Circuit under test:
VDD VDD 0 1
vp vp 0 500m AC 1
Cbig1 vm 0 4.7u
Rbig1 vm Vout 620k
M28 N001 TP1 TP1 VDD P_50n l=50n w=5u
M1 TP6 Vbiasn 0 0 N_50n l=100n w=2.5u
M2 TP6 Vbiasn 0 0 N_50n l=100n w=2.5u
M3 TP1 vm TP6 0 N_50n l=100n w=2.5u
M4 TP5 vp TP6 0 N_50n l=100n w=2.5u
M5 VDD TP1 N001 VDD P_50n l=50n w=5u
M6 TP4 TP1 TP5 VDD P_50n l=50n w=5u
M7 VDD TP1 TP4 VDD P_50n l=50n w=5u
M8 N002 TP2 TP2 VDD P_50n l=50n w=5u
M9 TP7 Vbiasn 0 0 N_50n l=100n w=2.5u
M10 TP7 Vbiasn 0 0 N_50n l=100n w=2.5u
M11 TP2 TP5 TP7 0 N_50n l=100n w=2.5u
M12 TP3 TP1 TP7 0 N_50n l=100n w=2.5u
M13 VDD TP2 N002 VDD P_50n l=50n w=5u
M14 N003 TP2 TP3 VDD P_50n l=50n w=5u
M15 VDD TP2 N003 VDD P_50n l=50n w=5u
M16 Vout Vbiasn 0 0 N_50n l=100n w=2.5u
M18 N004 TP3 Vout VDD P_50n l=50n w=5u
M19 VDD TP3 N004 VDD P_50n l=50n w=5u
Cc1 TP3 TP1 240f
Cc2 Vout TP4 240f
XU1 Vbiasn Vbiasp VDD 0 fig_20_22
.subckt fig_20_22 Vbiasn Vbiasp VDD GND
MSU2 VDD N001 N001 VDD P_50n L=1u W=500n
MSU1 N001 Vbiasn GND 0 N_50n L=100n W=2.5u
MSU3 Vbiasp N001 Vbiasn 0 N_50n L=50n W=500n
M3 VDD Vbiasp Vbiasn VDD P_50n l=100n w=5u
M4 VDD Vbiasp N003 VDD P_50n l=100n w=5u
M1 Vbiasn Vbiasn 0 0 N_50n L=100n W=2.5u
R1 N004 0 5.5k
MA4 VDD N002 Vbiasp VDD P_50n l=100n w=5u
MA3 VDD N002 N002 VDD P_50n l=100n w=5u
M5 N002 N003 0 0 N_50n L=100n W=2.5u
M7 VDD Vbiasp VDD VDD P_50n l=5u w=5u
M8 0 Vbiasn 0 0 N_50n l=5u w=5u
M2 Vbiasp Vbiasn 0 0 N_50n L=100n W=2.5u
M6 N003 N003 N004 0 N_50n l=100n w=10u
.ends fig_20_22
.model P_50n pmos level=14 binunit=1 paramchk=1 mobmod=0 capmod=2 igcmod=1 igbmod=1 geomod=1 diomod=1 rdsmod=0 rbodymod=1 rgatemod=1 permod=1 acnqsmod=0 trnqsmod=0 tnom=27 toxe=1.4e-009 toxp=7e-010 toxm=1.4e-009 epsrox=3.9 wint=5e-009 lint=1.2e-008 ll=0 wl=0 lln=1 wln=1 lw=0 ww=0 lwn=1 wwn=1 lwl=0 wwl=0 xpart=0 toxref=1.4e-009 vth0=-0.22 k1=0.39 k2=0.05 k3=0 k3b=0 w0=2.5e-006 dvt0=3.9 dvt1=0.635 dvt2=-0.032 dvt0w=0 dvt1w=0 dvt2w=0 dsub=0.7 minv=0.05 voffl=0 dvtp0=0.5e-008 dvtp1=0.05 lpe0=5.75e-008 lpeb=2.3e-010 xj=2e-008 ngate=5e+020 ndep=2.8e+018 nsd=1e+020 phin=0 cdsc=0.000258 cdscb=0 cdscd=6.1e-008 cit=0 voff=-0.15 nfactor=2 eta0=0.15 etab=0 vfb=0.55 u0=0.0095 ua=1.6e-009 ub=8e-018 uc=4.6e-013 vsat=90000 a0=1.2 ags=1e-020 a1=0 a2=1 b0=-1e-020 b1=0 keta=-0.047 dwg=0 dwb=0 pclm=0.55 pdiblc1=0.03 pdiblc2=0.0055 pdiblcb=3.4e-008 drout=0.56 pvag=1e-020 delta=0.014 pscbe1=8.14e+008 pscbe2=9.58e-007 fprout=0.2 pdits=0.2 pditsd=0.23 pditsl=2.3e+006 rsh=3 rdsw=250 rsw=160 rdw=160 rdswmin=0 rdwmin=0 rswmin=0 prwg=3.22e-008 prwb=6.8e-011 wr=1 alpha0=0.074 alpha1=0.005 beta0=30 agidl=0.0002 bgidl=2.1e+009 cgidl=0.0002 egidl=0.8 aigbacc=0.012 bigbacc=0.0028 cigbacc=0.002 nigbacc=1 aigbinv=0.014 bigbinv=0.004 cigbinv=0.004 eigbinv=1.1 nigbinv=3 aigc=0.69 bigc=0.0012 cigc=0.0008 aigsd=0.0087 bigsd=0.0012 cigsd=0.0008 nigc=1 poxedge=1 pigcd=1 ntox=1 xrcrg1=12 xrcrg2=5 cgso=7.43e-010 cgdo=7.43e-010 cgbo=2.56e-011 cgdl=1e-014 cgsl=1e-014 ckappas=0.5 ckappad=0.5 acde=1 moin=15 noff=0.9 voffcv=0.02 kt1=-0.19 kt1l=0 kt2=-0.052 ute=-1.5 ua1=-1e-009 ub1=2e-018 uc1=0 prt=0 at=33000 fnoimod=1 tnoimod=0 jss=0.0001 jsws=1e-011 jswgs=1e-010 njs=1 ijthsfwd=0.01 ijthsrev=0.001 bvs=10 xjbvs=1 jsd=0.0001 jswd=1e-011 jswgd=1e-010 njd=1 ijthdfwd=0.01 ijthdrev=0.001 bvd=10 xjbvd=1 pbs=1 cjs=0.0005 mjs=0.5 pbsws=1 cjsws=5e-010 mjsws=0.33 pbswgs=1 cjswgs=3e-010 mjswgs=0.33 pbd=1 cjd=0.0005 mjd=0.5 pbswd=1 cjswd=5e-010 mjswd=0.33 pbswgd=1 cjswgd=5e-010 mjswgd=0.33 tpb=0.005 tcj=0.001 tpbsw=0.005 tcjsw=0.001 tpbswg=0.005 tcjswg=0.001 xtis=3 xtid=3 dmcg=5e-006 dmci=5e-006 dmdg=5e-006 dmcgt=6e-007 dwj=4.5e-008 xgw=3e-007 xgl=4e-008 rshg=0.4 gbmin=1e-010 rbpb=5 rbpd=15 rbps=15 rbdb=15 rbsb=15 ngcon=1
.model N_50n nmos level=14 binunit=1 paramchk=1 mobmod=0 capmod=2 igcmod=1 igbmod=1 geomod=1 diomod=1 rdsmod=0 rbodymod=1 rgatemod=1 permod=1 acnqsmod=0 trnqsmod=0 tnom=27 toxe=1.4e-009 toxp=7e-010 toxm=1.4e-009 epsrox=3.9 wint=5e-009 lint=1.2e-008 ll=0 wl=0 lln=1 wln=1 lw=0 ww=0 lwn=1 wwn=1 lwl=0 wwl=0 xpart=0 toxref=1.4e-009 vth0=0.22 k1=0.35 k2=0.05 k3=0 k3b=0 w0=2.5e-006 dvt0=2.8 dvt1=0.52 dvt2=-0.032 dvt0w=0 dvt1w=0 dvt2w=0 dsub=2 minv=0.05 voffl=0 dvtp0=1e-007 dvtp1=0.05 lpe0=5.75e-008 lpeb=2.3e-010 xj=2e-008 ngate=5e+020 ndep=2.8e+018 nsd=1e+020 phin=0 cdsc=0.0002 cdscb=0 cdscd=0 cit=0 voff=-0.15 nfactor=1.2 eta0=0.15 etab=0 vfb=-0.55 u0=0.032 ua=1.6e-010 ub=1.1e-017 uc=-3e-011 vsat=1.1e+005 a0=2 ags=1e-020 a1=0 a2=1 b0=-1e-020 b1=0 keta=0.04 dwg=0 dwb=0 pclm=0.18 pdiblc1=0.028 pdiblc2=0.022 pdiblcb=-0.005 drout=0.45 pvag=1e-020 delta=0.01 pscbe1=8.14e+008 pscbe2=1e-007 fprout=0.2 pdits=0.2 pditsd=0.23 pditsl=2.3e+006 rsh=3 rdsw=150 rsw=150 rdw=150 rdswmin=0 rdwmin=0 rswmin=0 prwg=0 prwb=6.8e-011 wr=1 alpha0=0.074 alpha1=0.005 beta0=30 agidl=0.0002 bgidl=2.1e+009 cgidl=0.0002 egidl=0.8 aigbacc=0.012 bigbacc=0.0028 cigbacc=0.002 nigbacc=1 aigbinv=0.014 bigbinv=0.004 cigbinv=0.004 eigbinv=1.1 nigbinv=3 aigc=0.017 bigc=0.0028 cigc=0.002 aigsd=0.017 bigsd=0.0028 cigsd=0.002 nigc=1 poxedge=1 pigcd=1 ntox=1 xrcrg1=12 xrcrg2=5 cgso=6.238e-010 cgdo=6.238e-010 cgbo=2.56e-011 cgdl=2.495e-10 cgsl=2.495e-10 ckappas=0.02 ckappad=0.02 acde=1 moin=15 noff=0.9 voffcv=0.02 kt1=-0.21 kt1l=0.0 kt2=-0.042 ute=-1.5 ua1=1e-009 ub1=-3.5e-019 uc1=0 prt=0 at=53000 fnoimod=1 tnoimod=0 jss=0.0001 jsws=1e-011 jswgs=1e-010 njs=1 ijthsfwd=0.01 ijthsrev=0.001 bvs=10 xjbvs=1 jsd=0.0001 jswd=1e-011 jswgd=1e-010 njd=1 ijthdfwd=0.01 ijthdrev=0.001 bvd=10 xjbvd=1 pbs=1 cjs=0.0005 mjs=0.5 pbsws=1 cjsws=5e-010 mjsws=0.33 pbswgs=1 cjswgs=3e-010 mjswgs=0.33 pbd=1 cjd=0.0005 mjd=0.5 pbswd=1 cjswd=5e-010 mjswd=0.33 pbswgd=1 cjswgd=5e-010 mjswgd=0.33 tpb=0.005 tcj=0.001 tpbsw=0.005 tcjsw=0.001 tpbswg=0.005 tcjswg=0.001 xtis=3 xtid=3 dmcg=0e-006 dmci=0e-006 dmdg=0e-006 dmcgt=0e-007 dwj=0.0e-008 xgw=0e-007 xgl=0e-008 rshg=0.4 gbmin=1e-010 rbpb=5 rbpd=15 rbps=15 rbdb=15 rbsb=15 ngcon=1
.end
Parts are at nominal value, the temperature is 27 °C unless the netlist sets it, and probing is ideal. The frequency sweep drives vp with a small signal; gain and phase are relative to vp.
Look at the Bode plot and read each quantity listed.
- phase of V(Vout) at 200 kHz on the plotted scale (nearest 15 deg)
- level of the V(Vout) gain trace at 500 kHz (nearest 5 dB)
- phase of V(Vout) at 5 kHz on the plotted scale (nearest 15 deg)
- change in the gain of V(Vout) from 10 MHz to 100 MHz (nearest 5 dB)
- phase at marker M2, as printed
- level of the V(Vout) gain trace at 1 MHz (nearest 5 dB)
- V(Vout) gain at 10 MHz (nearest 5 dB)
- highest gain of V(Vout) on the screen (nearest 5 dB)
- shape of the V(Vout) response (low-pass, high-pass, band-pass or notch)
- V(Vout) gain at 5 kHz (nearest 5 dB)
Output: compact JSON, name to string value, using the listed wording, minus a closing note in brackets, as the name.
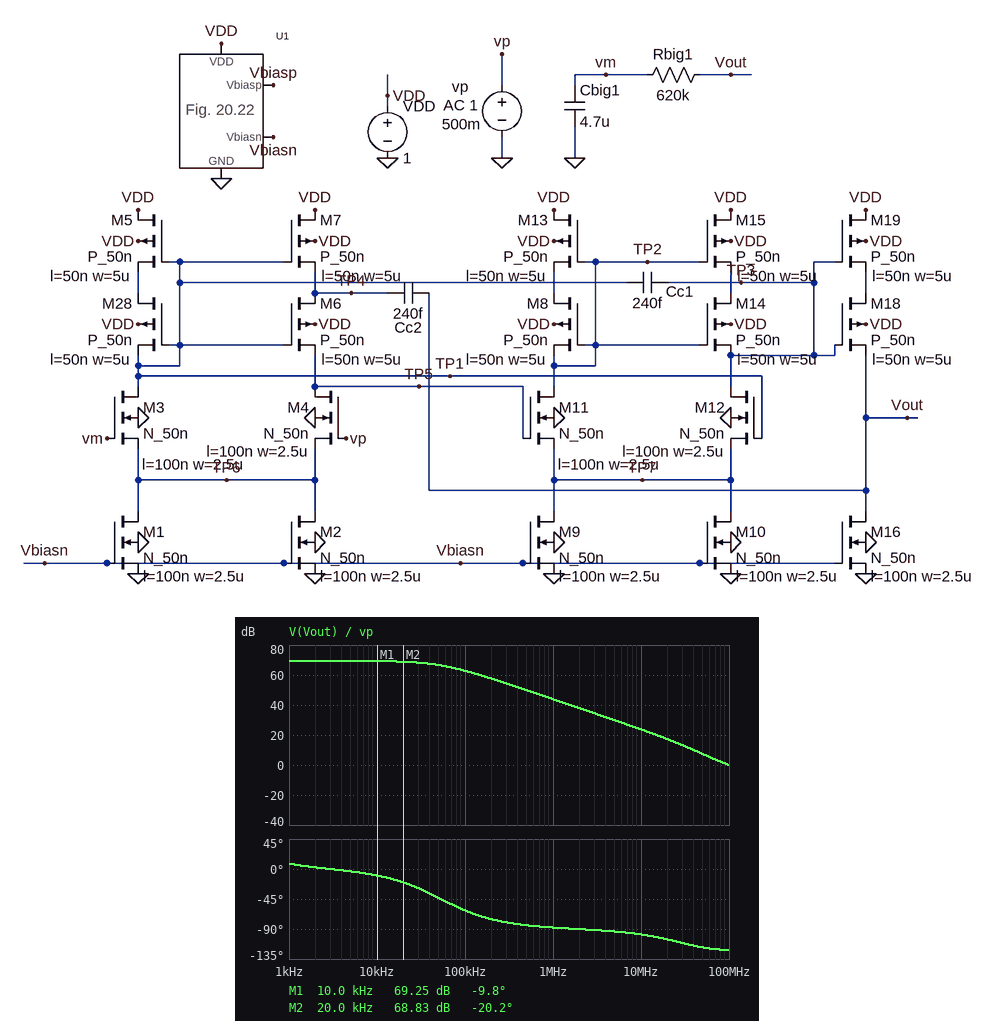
{"phase of V(Vout) at 200 kHz on the plotted scale": "-75 deg", "level of the V(Vout) gain trace at 500 kHz": "50 dB", "phase of V(Vout) at 5 kHz on the plotted scale": "0 deg", "change in the gain of V(Vout) from 10 MHz to 100 MHz": "-25 dB", "phase at marker M2, as printed": "-20.2 deg", "level of the V(Vout) gain trace at 1 MHz": "45 dB", "V(Vout) gain at 10 MHz": "25 dB", "highest gain of V(Vout) on the screen": "70 dB", "shape of the V(Vout) response": "low-pass", "V(Vout) gain at 5 kHz": "70 dB"}
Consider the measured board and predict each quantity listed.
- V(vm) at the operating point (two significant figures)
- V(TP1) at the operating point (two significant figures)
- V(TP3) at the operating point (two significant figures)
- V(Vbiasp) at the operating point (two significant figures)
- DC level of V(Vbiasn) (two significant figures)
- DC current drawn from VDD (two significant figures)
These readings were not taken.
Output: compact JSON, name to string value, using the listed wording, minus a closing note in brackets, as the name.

{"V(vm) at the operating point": "500 mV", "V(TP1) at the operating point": "680 mV", "V(TP3) at the operating point": "670 mV", "V(Vbiasp) at the operating point": "650 mV", "DC level of V(Vbiasn)": "350 mV", "DC current drawn from VDD": "96 µA"}
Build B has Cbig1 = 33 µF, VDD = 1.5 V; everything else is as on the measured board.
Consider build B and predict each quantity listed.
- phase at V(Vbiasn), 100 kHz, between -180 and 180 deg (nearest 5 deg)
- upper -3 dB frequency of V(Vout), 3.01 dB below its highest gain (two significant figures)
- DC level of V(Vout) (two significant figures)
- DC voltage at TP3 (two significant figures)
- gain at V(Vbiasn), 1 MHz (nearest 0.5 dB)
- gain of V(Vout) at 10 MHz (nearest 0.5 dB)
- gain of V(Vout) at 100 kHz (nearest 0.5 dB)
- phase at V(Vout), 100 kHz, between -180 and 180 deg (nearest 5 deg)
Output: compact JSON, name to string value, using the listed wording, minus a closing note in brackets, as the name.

{"phase at V(Vbiasn), 100 kHz, between -180 and 180 deg": "20 deg", "upper -3 dB frequency of V(Vout), 3.01 dB below its highest gain": "46 kHz", "DC level of V(Vout)": "500 mV", "DC voltage at TP3": "1.2 V", "gain at V(Vbiasn), 1 MHz": "-33.0 dB", "gain of V(Vout) at 10 MHz": "24.0 dB", "gain of V(Vout) at 100 kHz": "63.5 dB", "phase at V(Vout), 100 kHz, between -180 and 180 deg": "-65 deg"}
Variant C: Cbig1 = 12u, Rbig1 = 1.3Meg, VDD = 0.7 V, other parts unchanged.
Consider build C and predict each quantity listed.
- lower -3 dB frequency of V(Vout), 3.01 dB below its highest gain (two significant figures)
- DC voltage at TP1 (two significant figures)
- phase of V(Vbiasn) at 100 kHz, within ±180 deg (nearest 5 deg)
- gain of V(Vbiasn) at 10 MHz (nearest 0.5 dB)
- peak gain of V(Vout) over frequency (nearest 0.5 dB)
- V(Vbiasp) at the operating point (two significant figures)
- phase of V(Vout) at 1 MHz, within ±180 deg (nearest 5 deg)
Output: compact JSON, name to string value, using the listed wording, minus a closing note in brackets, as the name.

{"lower -3 dB frequency of V(Vout), 3.01 dB below its highest gain": "22 Hz", "DC voltage at TP1": "380 mV", "phase of V(Vbiasn) at 100 kHz, within ±180 deg": "30 deg", "gain of V(Vbiasn) at 10 MHz": "-35.5 dB", "peak gain of V(Vout) over frequency": "66.5 dB", "V(Vbiasp) at the operating point": "350 mV", "phase of V(Vout) at 1 MHz, within ±180 deg": "-85 deg"}
